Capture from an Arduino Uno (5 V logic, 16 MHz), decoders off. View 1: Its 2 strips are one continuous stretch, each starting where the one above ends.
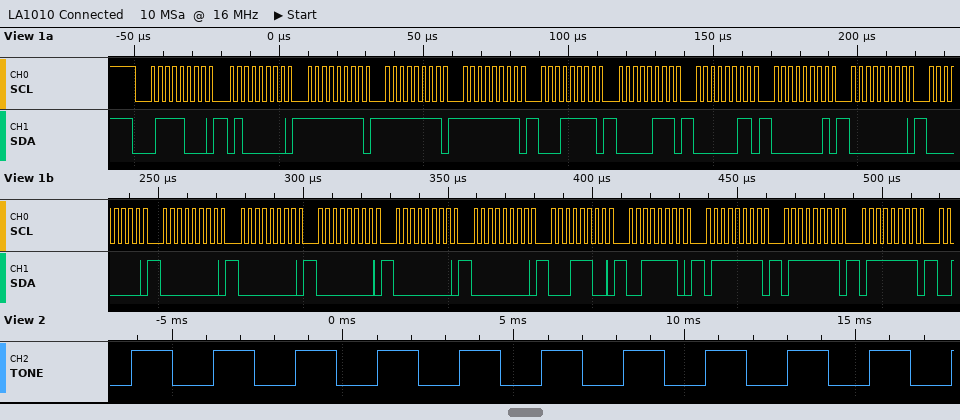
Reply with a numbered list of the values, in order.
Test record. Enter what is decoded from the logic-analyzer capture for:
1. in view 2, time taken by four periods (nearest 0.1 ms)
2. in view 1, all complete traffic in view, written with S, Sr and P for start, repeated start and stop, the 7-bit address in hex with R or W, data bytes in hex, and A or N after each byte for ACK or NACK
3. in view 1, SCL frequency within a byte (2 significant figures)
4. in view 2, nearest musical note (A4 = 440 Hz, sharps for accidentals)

1. 9.7 ms
2. S 3CW A 40 A FF A FF A FF A 1F A 07 A 03 A 01 A 00 A 00 A 00 A 00 A 00 A 00 A 00 A 1C A 3E A 7F A 7F A 7F A
3. 400 kHz
4. G#4
